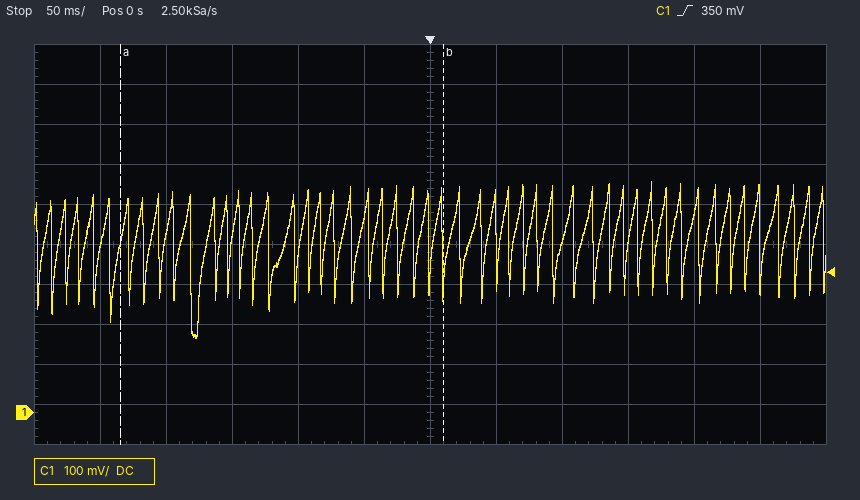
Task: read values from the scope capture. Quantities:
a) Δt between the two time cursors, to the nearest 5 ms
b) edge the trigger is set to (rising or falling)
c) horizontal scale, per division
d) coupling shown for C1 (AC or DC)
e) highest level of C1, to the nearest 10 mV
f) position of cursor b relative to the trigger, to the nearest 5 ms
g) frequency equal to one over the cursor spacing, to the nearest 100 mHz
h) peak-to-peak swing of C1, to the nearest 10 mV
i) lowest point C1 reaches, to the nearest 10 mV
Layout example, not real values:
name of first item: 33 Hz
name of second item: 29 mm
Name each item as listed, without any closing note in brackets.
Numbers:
Δt between the two time cursors, to the nearest 5 ms: 245 ms
edge the trigger is set to: rising
horizontal scale, per division: 50 ms
coupling shown for C1: DC
highest level of C1, to the nearest 10 mV: 580 mV
position of cursor b relative to the trigger, to the nearest 5 ms: +10 ms
frequency equal to one over the cursor spacing, to the nearest 100 mHz: 4.1 Hz
peak-to-peak swing of C1, to the nearest 10 mV: 390 mV
lowest point C1 reaches, to the nearest 10 mV: 190 mV
